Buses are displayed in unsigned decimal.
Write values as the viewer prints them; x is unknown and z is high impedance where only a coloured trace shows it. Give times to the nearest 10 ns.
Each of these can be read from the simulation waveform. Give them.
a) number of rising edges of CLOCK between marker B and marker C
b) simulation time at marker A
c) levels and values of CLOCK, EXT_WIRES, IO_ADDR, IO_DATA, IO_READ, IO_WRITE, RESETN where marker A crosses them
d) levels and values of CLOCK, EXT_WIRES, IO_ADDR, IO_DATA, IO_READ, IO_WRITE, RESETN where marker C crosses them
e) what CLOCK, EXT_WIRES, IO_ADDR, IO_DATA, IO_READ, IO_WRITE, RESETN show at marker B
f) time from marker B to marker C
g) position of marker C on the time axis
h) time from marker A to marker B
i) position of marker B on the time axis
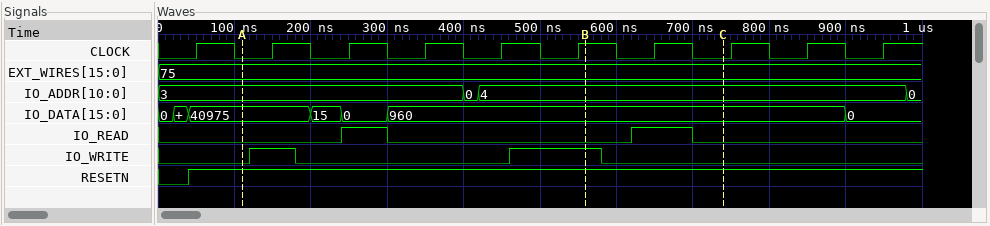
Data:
1
110 ns
CLOCK=0, EXT_WIRES=75, IO_ADDR=3, IO_DATA=40975, IO_READ=0, IO_WRITE=0, RESETN=1
CLOCK=0, EXT_WIRES=75, IO_ADDR=4, IO_DATA=960, IO_READ=0, IO_WRITE=0, RESETN=1
CLOCK=1, EXT_WIRES=75, IO_ADDR=4, IO_DATA=960, IO_READ=0, IO_WRITE=1, RESETN=1
180 ns
740 ns
450 ns
560 ns
